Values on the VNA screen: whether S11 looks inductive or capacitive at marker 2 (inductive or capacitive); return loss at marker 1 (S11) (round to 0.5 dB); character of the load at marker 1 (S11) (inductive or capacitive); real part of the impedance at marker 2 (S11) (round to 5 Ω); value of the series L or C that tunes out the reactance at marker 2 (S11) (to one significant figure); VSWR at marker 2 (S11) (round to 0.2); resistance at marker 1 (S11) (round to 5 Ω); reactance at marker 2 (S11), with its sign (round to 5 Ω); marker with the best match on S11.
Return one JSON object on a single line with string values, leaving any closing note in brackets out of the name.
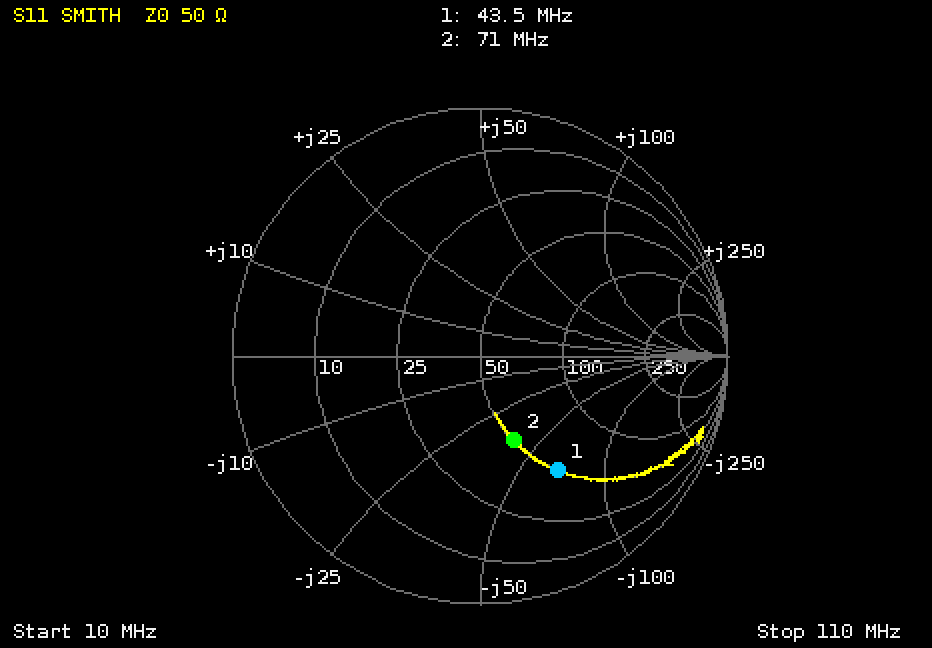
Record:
{"whether S11 looks inductive or capacitive at marker 2": "capacitive", "return loss at marker 1 (S11)": "5.0 dB", "character of the load at marker 1 (S11)": "capacitive", "real part of the impedance at marker 2 (S11)": "50 Ω", "value of the series L or C that tunes out the reactance at marker 2 (S11)": "90 nH", "VSWR at marker 2 (S11)": "2.2", "resistance at marker 1 (S11)": "50 Ω", "reactance at marker 2 (S11), with its sign": "-40 Ω", "marker with the best match on S11": "marker 2"}
